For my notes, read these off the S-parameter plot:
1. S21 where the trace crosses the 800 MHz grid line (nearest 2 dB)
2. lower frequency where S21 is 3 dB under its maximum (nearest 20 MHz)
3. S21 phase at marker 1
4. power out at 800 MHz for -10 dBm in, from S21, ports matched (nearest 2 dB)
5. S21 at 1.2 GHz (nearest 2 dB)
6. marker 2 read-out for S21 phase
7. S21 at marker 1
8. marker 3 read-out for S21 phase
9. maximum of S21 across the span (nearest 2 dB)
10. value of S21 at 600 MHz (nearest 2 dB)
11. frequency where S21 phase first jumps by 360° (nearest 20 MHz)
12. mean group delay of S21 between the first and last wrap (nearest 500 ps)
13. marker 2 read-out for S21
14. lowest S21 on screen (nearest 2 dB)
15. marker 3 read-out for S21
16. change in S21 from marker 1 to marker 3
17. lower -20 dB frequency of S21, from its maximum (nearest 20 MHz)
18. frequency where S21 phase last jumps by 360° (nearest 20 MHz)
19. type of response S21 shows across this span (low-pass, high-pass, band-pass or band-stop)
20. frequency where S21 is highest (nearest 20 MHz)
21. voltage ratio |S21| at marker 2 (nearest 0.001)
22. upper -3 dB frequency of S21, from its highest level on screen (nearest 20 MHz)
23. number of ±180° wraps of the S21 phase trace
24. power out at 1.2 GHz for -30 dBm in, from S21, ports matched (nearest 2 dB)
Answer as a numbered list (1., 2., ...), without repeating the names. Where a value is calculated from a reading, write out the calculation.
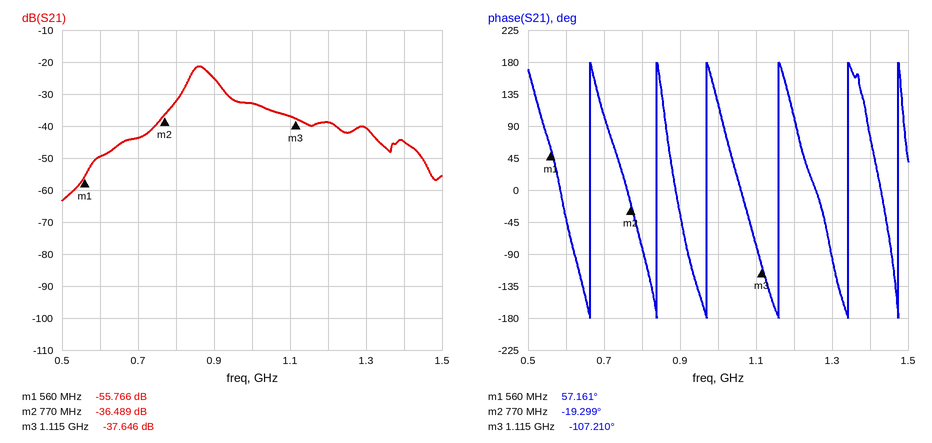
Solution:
1. -32 dB
2. 840 MHz
3. 57.161°
4. -10 dBm + (-32 dB) = -42 dBm
5. -38 dB
6. -19.299°
7. -55.766 dB
8. -107.210°
9. -22 dB
10. -50 dB
11. 660 MHz
12. 5 cycles / (1.48 GHz − 660 MHz) ≈ 6.10 ns, so 6.0 ns to the nearest 500 ps
13. -36.489 dB
14. -64 dB
15. -37.646 dB
16. -37.646 − (-55.766) = 18.120 dB
17. 740 MHz
18. 1.48 GHz
19. band-pass
20. 860 MHz
21. 10^(-36.489/20) ≈ 0.015
22. 900 MHz
23. 6
24. -30 dBm + (-38 dB) = -68 dBm
